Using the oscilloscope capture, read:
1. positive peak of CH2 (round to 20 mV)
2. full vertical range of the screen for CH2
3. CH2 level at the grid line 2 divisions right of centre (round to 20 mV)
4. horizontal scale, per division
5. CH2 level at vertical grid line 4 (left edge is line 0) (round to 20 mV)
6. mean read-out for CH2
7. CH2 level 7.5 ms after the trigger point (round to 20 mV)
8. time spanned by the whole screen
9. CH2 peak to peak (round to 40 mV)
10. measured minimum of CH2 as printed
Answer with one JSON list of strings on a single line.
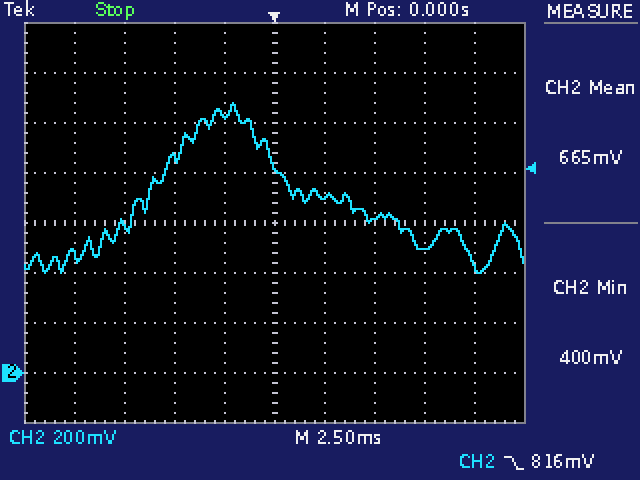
["1.08 V", "1.6 V", "620 mV", "2.5 ms", "1.04 V", "665 mV", "500 mV", "25 ms", "680 mV", "400 mV"]
